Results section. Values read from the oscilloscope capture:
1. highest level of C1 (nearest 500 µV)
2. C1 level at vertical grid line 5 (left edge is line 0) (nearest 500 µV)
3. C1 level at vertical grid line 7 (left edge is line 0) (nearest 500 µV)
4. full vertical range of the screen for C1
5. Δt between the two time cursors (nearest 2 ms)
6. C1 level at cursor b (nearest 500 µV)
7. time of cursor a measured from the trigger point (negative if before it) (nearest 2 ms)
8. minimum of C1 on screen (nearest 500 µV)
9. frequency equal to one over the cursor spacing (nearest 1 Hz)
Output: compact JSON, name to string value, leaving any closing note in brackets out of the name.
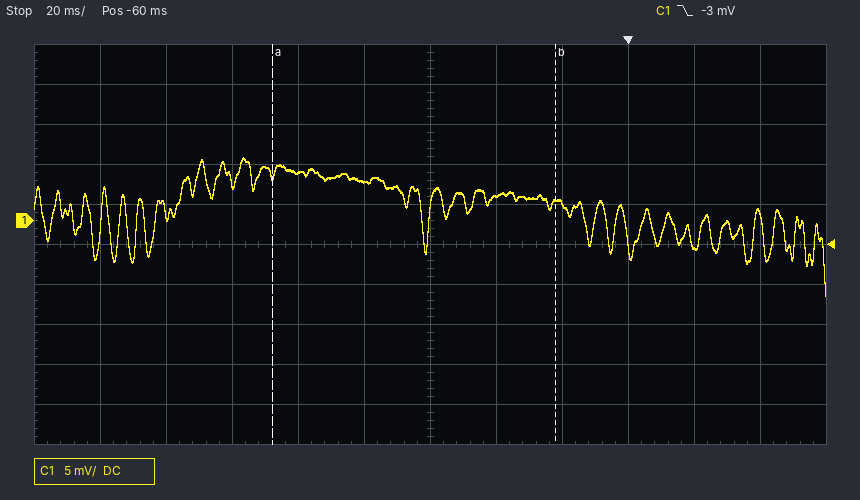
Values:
{"highest level of C1": "8.0 mV", "C1 level at vertical grid line 5 (left edge is line 0)": "5.0 mV", "C1 level at vertical grid line 7 (left edge is line 0)": "3.0 mV", "full vertical range of the screen for C1": "50 mV", "Δt between the two time cursors": "86 ms", "C1 level at cursor b": "2.5 mV", "time of cursor a measured from the trigger point (negative if before it)": "-108 ms", "minimum of C1 on screen": "-9.5 mV", "frequency equal to one over the cursor spacing": "12 Hz"}
